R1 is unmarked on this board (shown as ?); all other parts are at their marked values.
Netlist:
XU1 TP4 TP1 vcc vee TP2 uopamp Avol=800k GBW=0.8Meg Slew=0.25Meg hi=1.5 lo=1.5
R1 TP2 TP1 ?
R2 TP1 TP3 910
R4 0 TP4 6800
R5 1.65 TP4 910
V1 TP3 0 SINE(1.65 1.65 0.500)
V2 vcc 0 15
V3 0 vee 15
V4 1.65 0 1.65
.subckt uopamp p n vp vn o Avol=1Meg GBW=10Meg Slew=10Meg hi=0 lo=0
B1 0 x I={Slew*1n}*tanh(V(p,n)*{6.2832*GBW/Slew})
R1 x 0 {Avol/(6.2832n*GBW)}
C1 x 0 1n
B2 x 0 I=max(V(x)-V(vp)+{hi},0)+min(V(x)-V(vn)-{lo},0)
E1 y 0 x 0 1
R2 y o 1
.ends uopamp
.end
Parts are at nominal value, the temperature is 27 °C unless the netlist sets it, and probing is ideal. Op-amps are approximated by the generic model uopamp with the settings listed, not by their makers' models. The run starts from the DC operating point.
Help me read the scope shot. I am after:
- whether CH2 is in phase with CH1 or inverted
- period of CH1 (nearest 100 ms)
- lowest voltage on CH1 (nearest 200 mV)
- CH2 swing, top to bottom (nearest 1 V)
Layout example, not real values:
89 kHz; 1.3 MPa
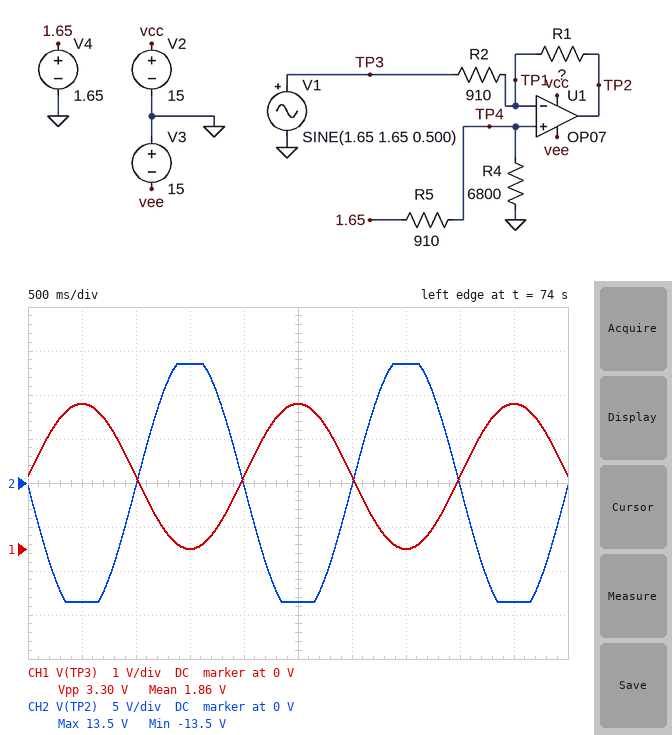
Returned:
inverted; 2.0 s; 0 V; 27 V
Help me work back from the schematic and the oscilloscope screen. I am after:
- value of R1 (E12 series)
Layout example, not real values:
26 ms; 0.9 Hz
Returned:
8.2 kΩ
